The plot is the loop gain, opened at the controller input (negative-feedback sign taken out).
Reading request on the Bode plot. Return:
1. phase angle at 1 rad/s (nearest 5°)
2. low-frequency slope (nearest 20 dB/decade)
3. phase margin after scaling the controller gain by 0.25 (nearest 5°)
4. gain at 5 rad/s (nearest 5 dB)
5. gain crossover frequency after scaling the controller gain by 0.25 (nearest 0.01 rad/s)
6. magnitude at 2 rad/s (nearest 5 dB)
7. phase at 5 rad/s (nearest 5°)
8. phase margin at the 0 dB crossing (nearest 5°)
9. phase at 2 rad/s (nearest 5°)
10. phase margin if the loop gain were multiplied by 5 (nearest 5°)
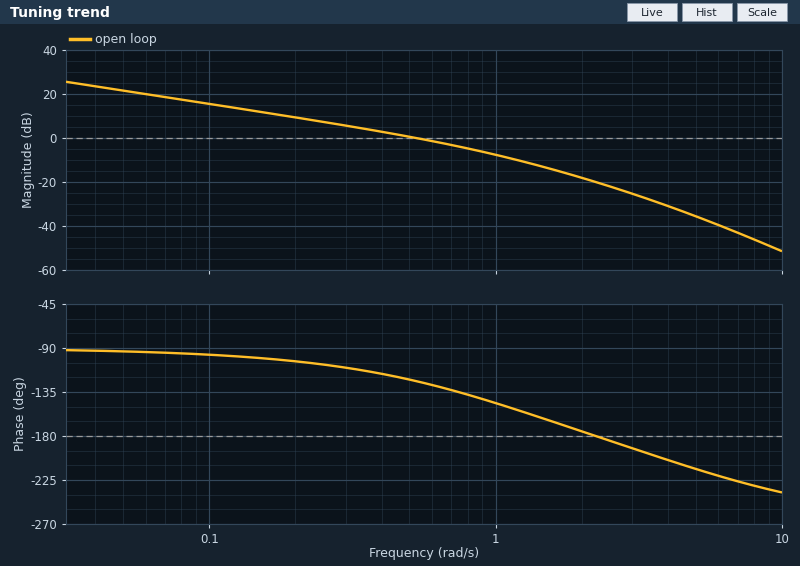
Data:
-145°
-20 dB/decade
80°
-35 dB
0.15 rad/s
-20 dB
-215°
55°
-175°
15°
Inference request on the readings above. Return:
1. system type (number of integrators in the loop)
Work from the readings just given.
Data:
1
